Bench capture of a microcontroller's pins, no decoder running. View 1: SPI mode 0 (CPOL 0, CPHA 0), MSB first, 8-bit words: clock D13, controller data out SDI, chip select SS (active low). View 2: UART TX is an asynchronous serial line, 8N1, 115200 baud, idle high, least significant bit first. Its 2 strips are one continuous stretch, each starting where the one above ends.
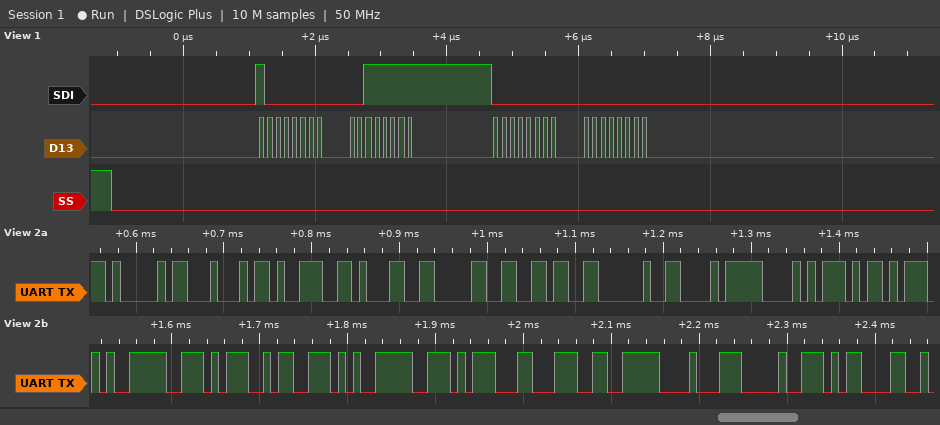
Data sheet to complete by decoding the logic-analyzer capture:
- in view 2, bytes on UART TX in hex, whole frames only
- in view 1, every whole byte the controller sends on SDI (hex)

0x41 0x44 0x39 0x31 0x30 0x36 0x20 0xE8 0xA8 0xAD 0xE5 0xAE 0x9A 0xE5 0xAE 0x8C 0xE6 0x88 0x90 0x0D
80 3F 00 00
